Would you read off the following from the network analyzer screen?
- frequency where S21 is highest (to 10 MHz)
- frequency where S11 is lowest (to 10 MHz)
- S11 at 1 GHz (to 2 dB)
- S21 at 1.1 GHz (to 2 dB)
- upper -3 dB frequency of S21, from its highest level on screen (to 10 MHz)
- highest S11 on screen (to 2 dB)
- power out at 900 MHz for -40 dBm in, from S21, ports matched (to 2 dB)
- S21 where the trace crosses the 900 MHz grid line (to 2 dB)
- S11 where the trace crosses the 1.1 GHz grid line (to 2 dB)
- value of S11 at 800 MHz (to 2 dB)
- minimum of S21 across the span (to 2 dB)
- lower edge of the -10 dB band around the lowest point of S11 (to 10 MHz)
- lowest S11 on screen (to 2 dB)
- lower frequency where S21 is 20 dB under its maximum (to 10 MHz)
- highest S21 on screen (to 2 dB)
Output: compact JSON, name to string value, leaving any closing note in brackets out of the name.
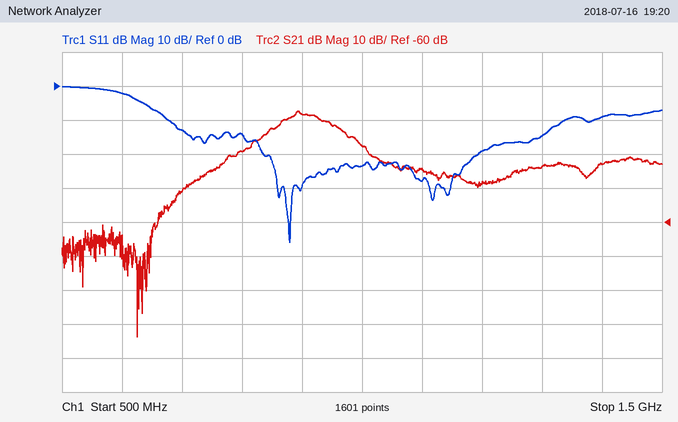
{"frequency where S21 is highest": "890 MHz", "frequency where S11 is lowest": "880 MHz", "S11 at 1 GHz": "-24 dB", "S21 at 1.1 GHz": "-44 dB", "upper -3 dB frequency of S21, from its highest level on screen": "940 MHz", "highest S11 on screen": "0 dB", "power out at 900 MHz for -40 dBm in, from S21, ports matched": "-68 dBm", "S21 where the trace crosses the 900 MHz grid line": "-28 dB", "S11 where the trace crosses the 1.1 GHz grid line": "-28 dB", "value of S11 at 800 MHz": "-14 dB", "minimum of S21 across the span": "-94 dB", "lower edge of the -10 dB band around the lowest point of S11": "680 MHz", "lowest S11 on screen": "-46 dB", "lower frequency where S21 is 20 dB under its maximum": "730 MHz", "highest S21 on screen": "-28 dB"}
